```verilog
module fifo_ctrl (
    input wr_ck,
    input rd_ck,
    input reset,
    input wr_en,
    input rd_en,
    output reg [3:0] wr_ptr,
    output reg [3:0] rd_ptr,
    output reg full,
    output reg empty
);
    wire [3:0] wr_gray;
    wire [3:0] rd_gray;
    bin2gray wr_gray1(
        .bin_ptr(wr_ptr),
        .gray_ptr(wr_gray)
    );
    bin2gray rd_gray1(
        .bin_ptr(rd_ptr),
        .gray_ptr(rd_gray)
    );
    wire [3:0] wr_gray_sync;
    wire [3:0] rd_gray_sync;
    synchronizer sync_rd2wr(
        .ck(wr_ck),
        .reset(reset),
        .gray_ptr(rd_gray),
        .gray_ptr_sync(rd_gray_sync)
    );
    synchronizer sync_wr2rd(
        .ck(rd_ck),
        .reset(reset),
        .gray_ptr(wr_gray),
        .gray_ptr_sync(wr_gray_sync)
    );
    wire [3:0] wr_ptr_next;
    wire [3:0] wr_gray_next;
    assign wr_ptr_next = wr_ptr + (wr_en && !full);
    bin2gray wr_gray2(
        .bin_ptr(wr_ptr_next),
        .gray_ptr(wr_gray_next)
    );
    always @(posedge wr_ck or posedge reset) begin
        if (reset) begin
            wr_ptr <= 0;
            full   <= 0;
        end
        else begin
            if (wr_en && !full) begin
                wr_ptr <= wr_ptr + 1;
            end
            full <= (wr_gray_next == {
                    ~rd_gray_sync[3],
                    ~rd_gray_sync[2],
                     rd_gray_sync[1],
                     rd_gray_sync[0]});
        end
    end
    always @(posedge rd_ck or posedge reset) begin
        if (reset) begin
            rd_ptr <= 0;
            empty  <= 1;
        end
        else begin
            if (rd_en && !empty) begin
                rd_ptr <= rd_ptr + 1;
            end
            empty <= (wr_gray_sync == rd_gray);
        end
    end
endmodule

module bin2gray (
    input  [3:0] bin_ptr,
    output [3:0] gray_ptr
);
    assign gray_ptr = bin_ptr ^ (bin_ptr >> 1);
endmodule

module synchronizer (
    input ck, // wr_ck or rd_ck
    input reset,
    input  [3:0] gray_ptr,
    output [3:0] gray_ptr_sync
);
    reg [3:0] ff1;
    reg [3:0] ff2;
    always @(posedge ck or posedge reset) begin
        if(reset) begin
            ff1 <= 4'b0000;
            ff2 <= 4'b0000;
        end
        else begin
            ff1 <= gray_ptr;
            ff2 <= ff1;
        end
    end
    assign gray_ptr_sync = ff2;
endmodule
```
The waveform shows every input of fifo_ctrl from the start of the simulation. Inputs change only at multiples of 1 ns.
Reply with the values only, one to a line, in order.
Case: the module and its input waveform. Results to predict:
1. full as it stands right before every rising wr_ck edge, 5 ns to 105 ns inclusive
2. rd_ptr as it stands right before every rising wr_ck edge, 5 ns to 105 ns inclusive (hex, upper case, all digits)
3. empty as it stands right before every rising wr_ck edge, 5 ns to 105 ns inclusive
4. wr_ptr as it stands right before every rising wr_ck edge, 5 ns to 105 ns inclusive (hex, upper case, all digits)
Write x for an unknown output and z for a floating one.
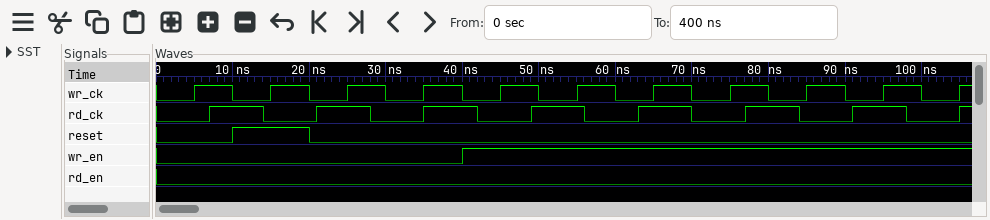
x 0 0 0 0 0 0 0 0 0 0
x, 0, 0, 0, 0, 0, 0, 0, 0, 0, 0
x 1 1 1 1 1 1 1 0 0 0
x, 0, 0, 0, 0, 1, 2, 3, 4, 5, 6
